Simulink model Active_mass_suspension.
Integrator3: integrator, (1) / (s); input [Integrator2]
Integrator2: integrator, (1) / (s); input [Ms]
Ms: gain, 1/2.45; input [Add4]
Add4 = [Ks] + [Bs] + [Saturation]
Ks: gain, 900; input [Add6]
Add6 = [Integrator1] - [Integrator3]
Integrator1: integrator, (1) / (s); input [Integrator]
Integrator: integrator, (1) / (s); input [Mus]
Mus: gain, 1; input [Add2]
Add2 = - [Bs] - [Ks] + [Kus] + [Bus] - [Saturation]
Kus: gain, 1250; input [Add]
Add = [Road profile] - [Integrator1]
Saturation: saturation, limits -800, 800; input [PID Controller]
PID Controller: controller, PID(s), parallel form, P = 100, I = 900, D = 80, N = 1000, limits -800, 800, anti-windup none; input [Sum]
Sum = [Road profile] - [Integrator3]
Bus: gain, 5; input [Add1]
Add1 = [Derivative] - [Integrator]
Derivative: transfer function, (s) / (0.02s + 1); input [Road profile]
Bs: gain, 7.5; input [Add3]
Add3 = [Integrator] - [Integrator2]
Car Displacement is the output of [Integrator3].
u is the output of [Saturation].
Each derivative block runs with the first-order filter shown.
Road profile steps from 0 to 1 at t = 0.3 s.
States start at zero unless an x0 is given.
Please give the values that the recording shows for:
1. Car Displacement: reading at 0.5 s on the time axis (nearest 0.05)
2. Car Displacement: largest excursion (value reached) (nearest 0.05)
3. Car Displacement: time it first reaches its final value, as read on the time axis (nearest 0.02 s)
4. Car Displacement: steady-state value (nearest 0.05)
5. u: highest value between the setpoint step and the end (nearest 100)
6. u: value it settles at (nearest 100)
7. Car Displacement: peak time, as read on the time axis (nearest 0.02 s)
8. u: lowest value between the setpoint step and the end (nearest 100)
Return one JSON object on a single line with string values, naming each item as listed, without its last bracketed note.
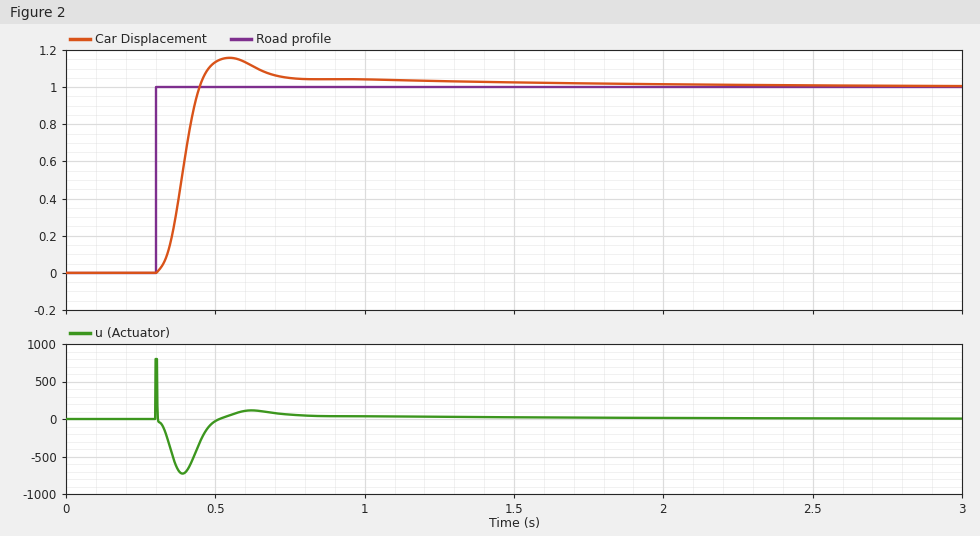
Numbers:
{"Car Displacement: reading at 0.5 s on the time axis": "1.15", "Car Displacement: largest excursion (value reached)": "1.15", "Car Displacement: time it first reaches its final value, as read on the time axis": "0.44 s", "Car Displacement: steady-state value": "1.00", "u: highest value between the setpoint step and the end": "800", "u: value it settles at": "0", "Car Displacement: peak time, as read on the time axis": "0.54 s", "u: lowest value between the setpoint step and the end": "-700"}
